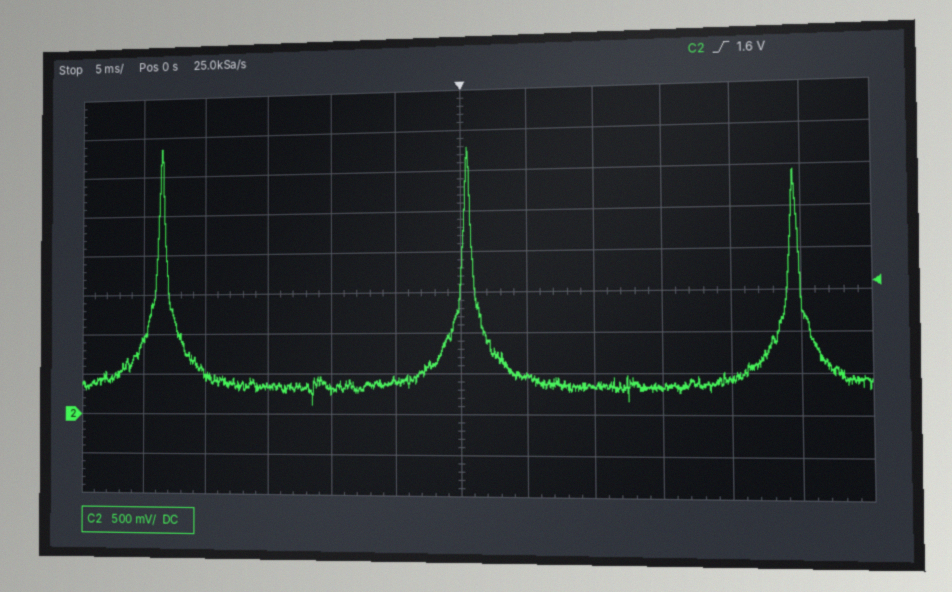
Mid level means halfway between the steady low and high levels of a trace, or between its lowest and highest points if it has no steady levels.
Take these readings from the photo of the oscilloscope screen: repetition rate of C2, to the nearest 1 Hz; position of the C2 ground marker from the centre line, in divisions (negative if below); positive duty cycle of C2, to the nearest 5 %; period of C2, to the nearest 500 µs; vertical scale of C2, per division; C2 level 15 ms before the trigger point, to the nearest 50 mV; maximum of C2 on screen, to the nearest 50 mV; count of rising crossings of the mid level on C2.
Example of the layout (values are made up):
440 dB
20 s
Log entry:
42 Hz
-3.0 div
5 %
24.0 ms
500 mV
350 mV
3.35 V
3
